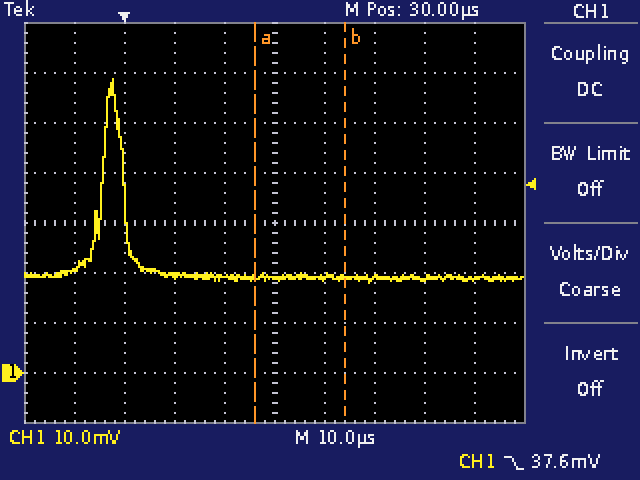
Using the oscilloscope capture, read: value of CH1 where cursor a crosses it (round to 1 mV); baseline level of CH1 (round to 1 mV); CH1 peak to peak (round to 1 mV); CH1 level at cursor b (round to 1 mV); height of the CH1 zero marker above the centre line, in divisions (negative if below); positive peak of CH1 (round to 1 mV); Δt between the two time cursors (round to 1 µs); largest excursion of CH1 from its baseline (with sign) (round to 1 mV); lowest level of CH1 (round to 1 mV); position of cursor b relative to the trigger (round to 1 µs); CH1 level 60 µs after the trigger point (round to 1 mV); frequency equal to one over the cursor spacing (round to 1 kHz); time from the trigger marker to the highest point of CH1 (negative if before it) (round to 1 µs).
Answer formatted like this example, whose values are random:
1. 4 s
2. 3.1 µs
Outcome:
1. 19 mV
2. 19 mV
3. 41 mV
4. 19 mV
5. -3.0 div
6. 59 mV
7. 18 µs
8. +40 mV
9. 18 mV
10. +44 µs
11. 19 mV
12. 56 kHz
13. -2 µs
